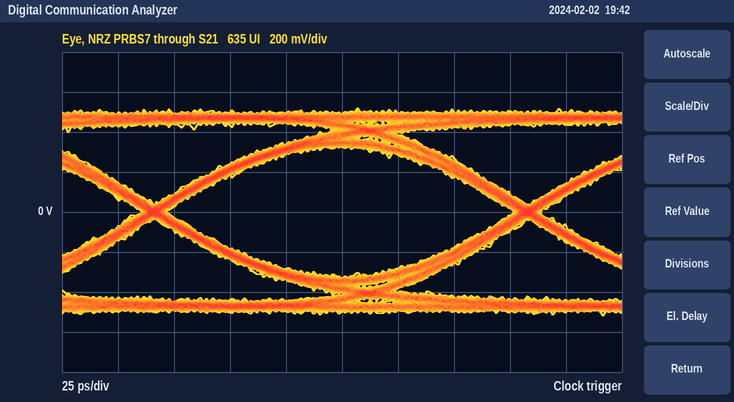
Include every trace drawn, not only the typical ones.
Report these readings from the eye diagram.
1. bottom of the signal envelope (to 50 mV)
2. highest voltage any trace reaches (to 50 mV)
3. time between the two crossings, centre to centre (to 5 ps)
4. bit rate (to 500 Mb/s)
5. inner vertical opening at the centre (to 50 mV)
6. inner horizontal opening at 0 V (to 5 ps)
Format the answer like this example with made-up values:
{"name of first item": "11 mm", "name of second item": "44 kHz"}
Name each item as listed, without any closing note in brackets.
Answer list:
{"bottom of the signal envelope": "-500 mV", "highest voltage any trace reaches": "500 mV", "time between the two crossings, centre to centre": "165 ps", "bit rate": "6.0 Gb/s", "inner vertical opening at the centre": "650 mV", "inner horizontal opening at 0 V": "155 ps"}
